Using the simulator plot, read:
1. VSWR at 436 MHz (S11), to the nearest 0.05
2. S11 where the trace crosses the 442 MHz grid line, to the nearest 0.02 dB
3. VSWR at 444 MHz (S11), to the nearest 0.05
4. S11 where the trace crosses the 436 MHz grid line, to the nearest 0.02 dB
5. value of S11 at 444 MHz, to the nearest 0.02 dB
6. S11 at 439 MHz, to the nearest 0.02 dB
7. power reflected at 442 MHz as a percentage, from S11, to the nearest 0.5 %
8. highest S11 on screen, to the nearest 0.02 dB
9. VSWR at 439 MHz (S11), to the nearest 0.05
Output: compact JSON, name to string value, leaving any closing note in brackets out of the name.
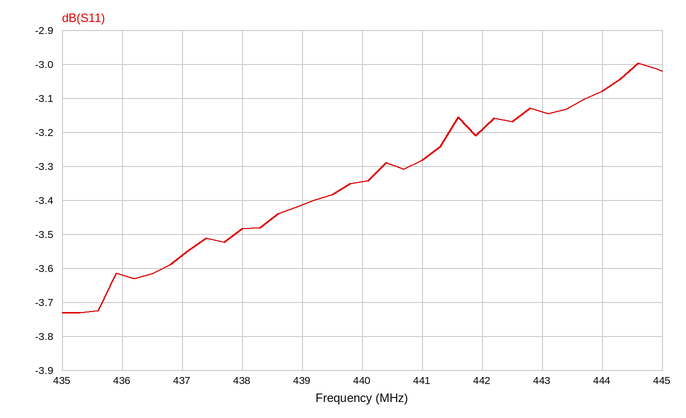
{"VSWR at 436 MHz (S11), to the nearest 0.05": "4.85", "S11 where the trace crosses the 442 MHz grid line, to the nearest 0.02 dB": "-3.20 dB", "VSWR at 444 MHz (S11), to the nearest 0.05": "5.70", "S11 where the trace crosses the 436 MHz grid line, to the nearest 0.02 dB": "-3.62 dB", "value of S11 at 444 MHz, to the nearest 0.02 dB": "-3.08 dB", "S11 at 439 MHz, to the nearest 0.02 dB": "-3.42 dB", "power reflected at 442 MHz as a percentage, from S11, to the nearest 0.5 %": "48.0 %", "highest S11 on screen, to the nearest 0.02 dB": "-3.00 dB", "VSWR at 439 MHz (S11), to the nearest 0.05": "5.15"}
